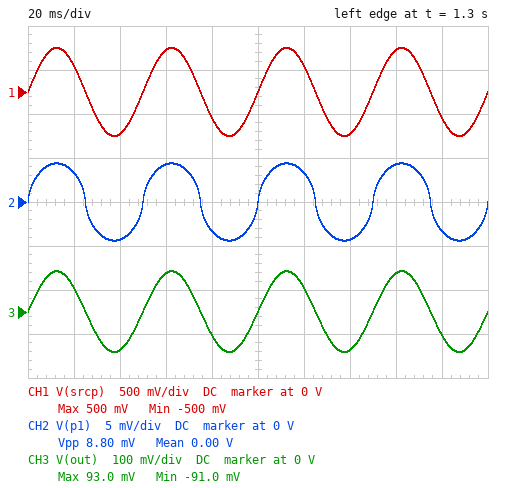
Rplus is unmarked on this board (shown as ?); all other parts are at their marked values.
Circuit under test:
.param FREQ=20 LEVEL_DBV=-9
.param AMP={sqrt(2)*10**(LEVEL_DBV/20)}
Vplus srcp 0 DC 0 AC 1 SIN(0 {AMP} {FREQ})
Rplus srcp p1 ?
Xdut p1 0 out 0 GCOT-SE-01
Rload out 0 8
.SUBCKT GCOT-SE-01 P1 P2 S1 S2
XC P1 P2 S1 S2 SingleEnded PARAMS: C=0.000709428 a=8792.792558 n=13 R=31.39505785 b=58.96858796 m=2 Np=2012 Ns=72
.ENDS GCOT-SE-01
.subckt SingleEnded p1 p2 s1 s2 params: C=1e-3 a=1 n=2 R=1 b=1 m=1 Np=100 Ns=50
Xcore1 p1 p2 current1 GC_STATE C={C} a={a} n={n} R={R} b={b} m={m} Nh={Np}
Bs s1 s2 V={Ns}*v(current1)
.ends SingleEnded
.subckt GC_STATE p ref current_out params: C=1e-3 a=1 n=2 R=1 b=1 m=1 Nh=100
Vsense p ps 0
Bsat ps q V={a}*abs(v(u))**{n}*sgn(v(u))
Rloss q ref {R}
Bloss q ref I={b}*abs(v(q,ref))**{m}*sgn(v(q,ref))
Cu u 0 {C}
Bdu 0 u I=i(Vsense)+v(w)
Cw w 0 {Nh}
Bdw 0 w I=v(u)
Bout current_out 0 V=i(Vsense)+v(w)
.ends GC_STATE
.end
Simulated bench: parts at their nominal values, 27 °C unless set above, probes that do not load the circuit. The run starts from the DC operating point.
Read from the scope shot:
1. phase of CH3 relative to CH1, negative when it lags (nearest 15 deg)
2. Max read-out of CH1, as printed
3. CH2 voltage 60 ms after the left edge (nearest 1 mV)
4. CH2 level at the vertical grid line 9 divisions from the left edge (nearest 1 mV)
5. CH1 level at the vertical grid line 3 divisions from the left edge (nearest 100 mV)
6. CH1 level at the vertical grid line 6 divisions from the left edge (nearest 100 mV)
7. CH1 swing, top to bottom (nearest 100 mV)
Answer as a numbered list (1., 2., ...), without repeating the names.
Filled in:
1. 0 deg
2. 500 mV
3. 4 mV
4. -3 mV
5. 500 mV
6. 300 mV
7. 1.0 V
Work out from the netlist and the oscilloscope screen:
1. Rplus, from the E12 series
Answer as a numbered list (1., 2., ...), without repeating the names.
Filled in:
1. 390 Ω
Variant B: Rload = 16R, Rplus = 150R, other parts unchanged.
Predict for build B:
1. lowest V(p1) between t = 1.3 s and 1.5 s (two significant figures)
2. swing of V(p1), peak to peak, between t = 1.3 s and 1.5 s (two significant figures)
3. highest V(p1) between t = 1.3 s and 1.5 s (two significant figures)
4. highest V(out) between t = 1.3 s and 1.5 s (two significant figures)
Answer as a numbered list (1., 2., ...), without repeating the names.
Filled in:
1. -7.2 mV
2. 14 mV
3. 7.2 mV
4. 240 mV
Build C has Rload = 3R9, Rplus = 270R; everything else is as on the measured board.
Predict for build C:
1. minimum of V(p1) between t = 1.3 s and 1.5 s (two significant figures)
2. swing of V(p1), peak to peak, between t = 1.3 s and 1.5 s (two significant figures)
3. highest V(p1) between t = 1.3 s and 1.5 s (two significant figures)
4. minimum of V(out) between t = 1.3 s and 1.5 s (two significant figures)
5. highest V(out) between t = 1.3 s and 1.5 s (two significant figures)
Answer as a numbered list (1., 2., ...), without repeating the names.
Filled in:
1. -5.3 mV
2. 11 mV
3. 5.3 mV
4. -130 mV
5. 130 mV
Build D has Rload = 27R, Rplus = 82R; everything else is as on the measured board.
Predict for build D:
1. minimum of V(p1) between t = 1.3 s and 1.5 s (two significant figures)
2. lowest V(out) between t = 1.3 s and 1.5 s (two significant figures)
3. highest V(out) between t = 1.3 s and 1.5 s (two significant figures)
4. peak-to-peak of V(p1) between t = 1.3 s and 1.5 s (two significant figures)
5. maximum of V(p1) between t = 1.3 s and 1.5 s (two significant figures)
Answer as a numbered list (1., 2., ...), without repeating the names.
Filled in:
1. -9.8 mV
2. -430 mV
3. 440 mV
4. 20 mV
5. 9.8 mV
